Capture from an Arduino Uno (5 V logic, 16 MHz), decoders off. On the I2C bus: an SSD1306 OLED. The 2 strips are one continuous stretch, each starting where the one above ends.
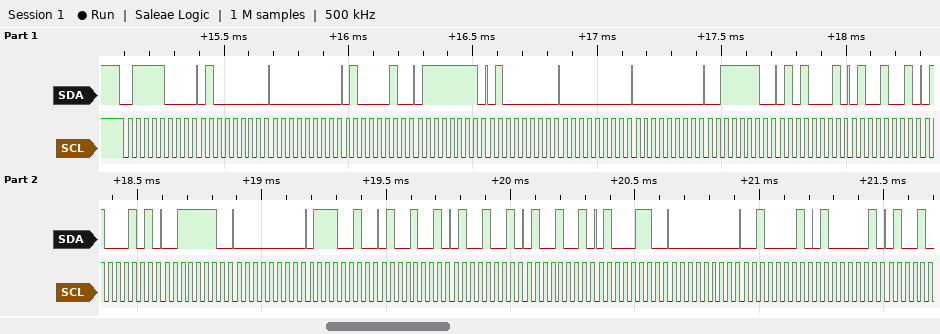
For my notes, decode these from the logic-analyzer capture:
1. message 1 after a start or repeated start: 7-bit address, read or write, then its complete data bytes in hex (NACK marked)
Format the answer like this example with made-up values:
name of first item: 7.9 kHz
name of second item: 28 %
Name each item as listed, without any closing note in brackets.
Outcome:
message 1 after a start or repeated start: 7-bit address, read or write, then its complete data bytes in hex: 0x3C write: 40 00 42 7F 40 00 00 3E 51 49 45 3E 00 72 49 49 49 46 00 21 41
